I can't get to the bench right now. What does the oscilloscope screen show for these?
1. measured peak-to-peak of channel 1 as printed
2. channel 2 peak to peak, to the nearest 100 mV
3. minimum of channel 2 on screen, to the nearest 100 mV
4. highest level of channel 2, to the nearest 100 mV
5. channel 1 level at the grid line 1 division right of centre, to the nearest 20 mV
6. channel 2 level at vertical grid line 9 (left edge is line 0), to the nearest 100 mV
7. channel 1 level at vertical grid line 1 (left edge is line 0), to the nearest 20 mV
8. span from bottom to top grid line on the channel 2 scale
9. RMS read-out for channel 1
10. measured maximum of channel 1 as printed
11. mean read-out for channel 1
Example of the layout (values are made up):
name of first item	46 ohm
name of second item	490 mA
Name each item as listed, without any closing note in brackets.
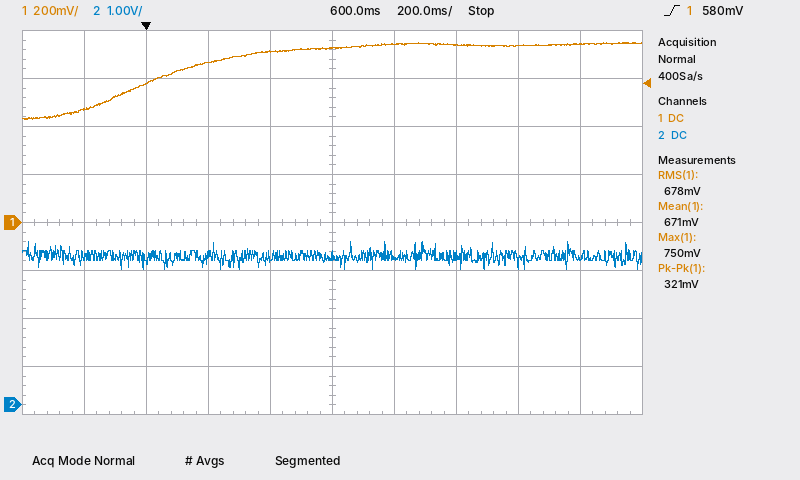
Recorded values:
measured peak-to-peak of channel 1 as printed	321 mV
channel 2 peak to peak, to the nearest 100 mV	600 mV
minimum of channel 2 on screen, to the nearest 100 mV	2.8 V
highest level of channel 2, to the nearest 100 mV	3.4 V
channel 1 level at the grid line 1 division right of centre, to the nearest 20 mV	740 mV
channel 2 level at vertical grid line 9 (left edge is line 0), to the nearest 100 mV	3.1 V
channel 1 level at vertical grid line 1 (left edge is line 0), to the nearest 20 mV	480 mV
span from bottom to top grid line on the channel 2 scale	8 V
RMS read-out for channel 1	678 mV
measured maximum of channel 1 as printed	750 mV
mean read-out for channel 1	671 mV
